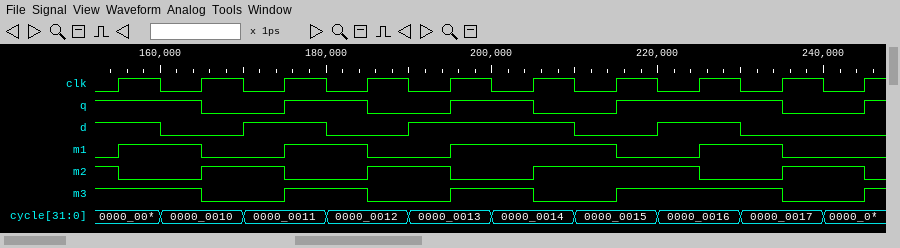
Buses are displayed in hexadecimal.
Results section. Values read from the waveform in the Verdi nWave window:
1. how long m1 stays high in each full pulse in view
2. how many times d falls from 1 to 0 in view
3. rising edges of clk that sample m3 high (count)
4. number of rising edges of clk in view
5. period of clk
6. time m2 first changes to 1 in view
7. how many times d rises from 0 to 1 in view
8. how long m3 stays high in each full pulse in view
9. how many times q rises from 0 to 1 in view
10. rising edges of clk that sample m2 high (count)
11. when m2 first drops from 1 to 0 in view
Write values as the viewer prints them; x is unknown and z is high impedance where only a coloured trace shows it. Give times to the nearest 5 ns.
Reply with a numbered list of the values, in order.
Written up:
1. 10 ns, 10 ns, 20 ns, 10 ns
2. 4
3. 6
4. 10
5. 10 ns
6. 165 ns
7. 3
8. 10 ns, 10 ns, 20 ns
9. 4
10. 6
11. 155 ns
